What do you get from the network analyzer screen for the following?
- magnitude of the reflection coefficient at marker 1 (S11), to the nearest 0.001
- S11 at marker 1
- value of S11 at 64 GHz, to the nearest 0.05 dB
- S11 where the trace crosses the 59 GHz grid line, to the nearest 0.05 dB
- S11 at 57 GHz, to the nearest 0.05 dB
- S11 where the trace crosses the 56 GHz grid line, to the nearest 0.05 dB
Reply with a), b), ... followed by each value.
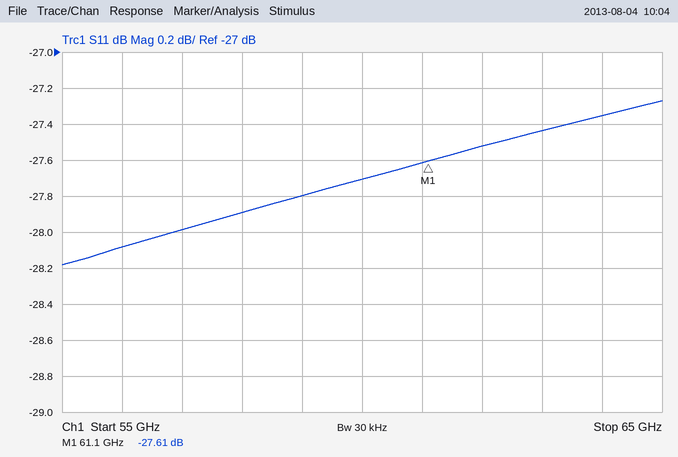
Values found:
a) 0.042
b) -27.61 dB
c) -27.35 dB
d) -27.80 dB
e) -28.00 dB
f) -28.10 dB
